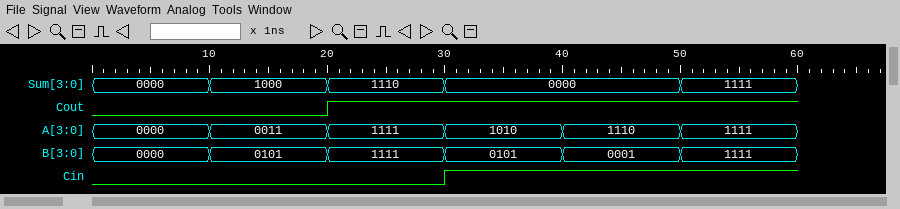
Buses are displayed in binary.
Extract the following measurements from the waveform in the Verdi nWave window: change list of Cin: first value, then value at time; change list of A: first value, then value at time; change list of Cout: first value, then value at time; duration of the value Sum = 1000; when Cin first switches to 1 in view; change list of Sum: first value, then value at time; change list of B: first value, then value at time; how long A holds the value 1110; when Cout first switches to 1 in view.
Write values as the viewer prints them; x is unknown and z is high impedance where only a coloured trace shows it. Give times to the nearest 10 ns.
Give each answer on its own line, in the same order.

0, 1 at 30 ns
0000, 0011 at 10 ns, 1111 at 20 ns, 1010 at 30 ns, 1110 at 40 ns, 1111 at 50 ns
0, 1 at 20 ns
10 ns
30 ns
0000, 1000 at 10 ns, 1110 at 20 ns, 0000 at 30 ns, 1111 at 50 ns
0000, 0101 at 10 ns, 1111 at 20 ns, 0101 at 30 ns, 0001 at 40 ns, 1111 at 50 ns
10 ns
20 ns
